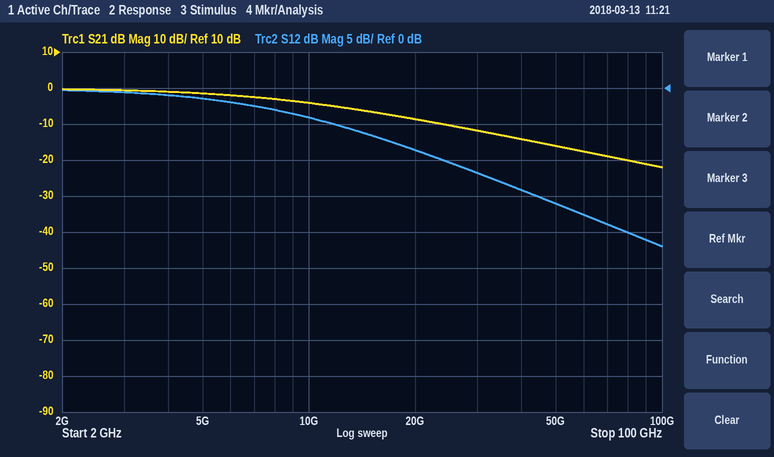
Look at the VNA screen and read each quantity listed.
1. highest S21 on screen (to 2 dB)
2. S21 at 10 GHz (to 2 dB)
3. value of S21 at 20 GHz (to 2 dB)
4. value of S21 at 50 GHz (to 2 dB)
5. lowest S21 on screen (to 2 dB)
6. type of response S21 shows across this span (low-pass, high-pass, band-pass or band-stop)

0 dB
-4 dB
-8 dB
-16 dB
-22 dB
low-pass
